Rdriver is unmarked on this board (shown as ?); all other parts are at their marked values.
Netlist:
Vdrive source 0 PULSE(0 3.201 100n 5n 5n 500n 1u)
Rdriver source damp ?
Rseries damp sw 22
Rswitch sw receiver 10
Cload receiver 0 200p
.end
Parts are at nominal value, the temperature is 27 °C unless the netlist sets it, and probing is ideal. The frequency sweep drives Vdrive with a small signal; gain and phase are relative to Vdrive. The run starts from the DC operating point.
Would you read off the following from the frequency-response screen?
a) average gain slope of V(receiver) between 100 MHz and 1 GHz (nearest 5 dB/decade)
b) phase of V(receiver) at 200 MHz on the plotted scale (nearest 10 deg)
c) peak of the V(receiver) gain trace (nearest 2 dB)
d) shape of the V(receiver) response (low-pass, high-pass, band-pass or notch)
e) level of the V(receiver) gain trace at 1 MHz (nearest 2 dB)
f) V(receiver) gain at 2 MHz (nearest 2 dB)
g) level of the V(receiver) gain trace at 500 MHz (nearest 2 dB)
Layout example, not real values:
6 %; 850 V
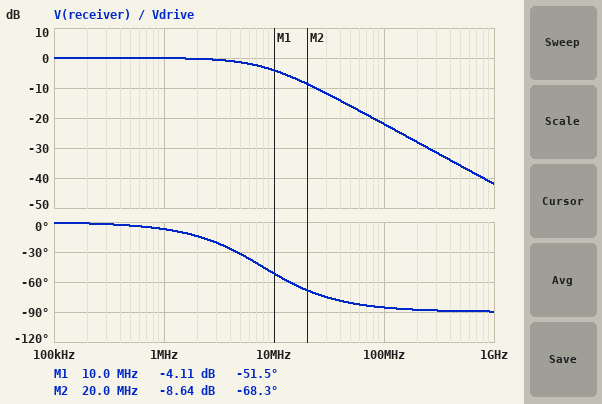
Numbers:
-20 dB/decade; -90 deg; 0 dB; low-pass; 0 dB; 0 dB; -36 dB
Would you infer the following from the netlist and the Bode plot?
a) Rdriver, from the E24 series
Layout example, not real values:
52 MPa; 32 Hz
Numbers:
68 Ω
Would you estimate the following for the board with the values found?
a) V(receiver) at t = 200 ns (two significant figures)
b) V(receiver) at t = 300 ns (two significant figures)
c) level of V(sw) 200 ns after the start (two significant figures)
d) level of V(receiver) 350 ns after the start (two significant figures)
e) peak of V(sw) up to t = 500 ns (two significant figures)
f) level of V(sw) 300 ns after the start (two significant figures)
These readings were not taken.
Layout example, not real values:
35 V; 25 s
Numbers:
3.2 V; 3.2 V; 3.2 V; 3.2 V; 3.2 V; 3.2 V
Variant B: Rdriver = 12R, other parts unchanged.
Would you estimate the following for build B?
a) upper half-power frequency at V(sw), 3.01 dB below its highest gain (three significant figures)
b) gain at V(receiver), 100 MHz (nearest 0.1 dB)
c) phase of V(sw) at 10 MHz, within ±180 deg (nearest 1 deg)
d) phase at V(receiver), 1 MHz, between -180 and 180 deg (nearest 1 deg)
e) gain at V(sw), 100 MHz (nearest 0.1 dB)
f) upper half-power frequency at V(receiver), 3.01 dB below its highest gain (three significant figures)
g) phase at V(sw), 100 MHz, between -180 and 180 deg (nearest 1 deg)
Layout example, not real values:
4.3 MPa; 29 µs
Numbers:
19.1 MHz; -15.0 dB; -22 deg; -3 deg; -10.9 dB; 18.1 MHz; -28 deg
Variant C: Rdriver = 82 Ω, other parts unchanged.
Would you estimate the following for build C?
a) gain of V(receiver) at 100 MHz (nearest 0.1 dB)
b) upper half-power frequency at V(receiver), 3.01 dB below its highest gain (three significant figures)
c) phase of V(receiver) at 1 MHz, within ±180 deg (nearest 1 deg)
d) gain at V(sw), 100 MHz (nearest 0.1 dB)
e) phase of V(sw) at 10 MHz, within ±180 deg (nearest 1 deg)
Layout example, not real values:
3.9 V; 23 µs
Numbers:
-23.1 dB; 6.98 MHz; -8 deg; -19.0 dB; -48 deg
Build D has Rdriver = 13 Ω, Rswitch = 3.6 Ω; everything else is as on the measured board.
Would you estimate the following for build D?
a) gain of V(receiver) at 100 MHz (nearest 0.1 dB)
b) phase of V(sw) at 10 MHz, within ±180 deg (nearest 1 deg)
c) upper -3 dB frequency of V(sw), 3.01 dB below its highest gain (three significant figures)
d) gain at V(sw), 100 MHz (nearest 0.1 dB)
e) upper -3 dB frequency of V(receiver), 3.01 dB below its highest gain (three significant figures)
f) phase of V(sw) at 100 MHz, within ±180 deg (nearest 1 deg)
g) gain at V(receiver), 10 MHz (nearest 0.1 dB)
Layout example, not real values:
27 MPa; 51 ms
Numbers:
-13.9 dB; -23 deg; 20.8 MHz; -13.1 dB; 20.6 MHz; -54 deg; -0.9 dB
